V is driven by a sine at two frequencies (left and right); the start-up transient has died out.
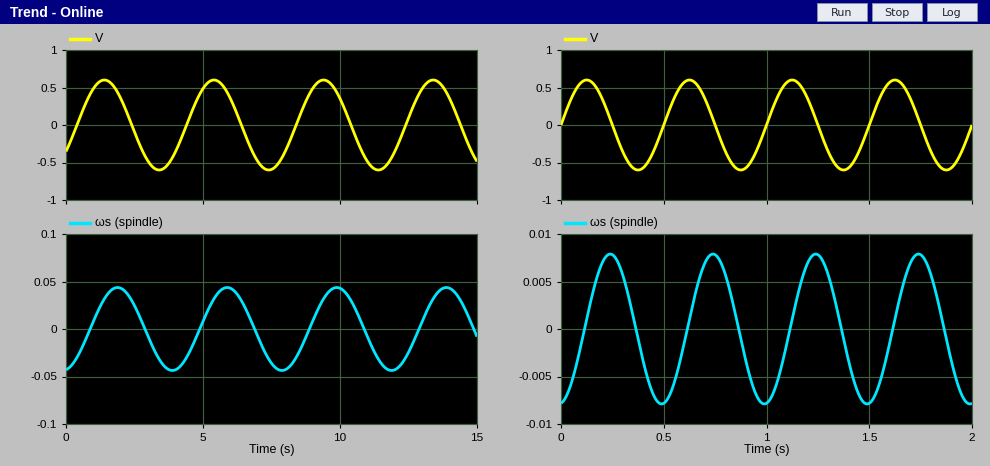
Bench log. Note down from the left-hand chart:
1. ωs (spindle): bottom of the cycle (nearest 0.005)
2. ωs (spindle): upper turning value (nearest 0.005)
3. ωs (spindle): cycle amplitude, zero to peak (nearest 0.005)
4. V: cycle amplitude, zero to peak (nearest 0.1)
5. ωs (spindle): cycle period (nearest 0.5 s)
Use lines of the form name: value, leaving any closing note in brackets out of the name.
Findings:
ωs (spindle): bottom of the cycle: -0.045
ωs (spindle): upper turning value: 0.045
ωs (spindle): cycle amplitude, zero to peak: 0.045
V: cycle amplitude, zero to peak: 0.6
ωs (spindle): cycle period: 4.0 s
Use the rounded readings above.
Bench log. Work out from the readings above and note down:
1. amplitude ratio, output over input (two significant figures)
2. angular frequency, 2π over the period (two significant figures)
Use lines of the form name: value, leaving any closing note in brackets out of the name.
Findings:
amplitude ratio, output over input: 0.075
angular frequency, 2π over the period: 1.6 rad/s
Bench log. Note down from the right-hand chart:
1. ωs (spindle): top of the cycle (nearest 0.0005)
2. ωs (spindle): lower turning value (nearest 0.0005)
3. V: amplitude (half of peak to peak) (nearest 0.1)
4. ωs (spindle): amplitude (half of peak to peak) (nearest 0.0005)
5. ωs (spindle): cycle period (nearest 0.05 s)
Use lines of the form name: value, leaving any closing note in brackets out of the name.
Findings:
ωs (spindle): top of the cycle: 0.0080
ωs (spindle): lower turning value: -0.0080
V: amplitude (half of peak to peak): 0.6
ωs (spindle): amplitude (half of peak to peak): 0.0080
ωs (spindle): cycle period: 0.50 s
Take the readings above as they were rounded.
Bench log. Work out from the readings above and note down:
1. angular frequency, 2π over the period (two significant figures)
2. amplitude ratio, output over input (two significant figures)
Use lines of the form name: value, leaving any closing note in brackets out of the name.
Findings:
angular frequency, 2π over the period: 13 rad/s
amplitude ratio, output over input: 0.013
